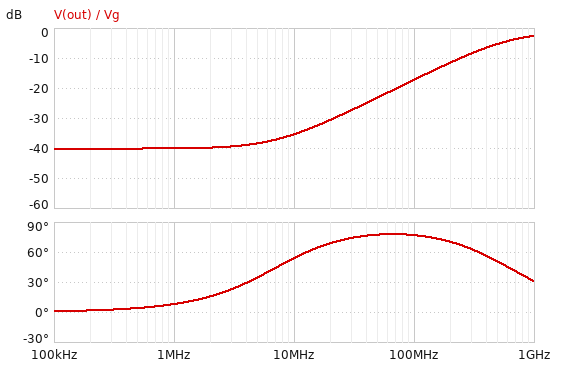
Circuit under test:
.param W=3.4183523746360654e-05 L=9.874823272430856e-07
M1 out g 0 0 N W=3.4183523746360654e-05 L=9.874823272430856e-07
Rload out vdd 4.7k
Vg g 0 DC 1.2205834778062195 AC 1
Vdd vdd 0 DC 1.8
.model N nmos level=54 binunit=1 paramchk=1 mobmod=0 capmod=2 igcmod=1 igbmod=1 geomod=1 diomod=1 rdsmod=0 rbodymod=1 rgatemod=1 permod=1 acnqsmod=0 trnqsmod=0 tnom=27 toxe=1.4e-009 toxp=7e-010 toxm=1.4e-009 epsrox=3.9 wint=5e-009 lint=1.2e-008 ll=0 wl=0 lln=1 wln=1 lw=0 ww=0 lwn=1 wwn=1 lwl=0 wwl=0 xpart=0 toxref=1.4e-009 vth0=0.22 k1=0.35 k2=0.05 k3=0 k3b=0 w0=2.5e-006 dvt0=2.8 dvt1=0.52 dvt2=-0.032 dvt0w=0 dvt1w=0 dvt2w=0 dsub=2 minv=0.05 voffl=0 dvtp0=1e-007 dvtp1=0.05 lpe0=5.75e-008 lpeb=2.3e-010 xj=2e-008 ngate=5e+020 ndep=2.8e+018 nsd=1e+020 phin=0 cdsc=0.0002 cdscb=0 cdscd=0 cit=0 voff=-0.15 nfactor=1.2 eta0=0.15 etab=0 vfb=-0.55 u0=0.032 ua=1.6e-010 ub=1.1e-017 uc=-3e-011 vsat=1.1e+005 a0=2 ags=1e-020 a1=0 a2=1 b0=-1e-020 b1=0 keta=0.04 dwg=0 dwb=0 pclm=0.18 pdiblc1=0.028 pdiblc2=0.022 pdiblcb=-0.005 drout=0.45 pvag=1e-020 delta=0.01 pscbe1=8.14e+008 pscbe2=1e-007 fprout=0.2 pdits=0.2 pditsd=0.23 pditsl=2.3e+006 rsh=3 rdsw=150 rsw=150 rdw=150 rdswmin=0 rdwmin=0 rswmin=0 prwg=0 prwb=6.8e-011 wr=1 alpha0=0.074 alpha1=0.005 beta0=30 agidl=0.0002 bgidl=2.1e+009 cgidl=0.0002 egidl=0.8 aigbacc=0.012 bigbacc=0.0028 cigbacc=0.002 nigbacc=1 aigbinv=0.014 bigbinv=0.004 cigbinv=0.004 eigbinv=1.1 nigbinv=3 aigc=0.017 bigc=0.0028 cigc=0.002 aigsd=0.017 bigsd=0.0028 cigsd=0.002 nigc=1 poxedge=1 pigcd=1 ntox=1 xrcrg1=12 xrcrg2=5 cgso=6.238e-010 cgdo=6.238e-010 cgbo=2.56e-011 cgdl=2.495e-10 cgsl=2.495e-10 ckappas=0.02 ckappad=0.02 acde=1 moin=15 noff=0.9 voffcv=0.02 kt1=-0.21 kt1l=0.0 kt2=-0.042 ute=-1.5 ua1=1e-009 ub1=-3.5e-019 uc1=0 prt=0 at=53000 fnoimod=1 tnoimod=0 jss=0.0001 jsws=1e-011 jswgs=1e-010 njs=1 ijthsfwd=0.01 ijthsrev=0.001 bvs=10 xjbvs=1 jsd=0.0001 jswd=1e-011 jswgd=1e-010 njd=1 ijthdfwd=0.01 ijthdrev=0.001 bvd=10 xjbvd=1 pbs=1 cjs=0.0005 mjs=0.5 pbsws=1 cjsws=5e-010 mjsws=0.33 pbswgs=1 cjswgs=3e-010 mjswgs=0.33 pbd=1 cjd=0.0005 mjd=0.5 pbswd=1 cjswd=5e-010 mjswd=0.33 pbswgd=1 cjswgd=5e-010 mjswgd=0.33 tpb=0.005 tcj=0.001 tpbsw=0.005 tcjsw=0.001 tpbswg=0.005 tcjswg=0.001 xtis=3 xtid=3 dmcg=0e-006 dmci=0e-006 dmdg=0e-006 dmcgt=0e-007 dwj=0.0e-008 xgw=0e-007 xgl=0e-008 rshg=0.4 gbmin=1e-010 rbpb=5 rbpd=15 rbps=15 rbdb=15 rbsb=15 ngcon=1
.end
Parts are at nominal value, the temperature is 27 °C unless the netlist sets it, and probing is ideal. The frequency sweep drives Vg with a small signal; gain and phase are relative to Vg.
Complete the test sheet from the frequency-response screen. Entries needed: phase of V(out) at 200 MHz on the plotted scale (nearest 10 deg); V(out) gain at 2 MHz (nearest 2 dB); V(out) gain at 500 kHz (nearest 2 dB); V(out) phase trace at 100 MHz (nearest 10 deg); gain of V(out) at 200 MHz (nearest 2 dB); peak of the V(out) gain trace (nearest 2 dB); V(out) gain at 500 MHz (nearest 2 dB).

70 deg
-40 dB
-40 dB
80 deg
-12 dB
-2 dB
-6 dB
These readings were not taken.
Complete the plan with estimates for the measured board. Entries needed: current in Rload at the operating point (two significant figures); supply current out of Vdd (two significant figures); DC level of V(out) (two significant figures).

360 µA
360 µA
110 mV
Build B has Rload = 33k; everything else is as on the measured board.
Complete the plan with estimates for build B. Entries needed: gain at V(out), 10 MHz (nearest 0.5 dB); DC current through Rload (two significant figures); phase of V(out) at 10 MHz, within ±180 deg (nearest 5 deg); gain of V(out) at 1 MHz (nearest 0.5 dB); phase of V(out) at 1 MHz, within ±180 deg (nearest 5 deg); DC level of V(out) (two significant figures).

-36.5 dB
54 µA
60 deg
-42.5 dB
10 deg
17 mV
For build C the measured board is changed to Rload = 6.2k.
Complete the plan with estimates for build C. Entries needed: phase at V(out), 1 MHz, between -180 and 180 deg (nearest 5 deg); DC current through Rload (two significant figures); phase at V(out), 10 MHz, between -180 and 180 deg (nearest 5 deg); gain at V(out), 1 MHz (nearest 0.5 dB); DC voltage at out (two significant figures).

5 deg
280 µA
50 deg
-39.5 dB
86 mV
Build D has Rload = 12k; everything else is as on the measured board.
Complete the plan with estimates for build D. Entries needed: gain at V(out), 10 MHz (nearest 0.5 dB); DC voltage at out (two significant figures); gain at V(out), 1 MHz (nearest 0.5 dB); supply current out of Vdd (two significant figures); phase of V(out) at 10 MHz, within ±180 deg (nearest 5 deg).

-36.0 dB
45 mV
-40.5 dB
150 µA
55 deg
